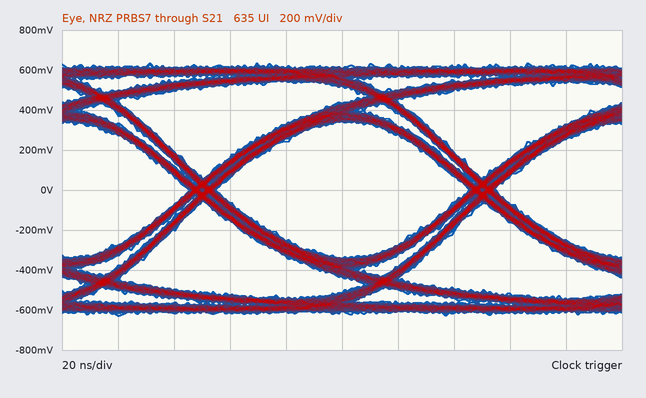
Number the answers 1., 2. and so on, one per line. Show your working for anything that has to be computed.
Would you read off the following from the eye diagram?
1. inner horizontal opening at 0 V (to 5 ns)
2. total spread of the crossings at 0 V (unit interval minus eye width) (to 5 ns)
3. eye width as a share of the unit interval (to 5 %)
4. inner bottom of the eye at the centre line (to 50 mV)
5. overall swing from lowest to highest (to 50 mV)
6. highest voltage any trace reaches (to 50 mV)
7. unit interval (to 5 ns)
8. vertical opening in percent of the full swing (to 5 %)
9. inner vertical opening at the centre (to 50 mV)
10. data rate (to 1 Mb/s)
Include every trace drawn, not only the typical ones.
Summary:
1. 90 ns
2. 10 ns
3. 90 ns / 100 ns ≈ 90 %
4. -350 mV
5. 1.25 V
6. 650 mV
7. 100 ns
8. 700 mV / 1.25 V ≈ 56.0 %, so 55 % to the nearest 5 %
9. 700 mV
10. 10 Mb/s
